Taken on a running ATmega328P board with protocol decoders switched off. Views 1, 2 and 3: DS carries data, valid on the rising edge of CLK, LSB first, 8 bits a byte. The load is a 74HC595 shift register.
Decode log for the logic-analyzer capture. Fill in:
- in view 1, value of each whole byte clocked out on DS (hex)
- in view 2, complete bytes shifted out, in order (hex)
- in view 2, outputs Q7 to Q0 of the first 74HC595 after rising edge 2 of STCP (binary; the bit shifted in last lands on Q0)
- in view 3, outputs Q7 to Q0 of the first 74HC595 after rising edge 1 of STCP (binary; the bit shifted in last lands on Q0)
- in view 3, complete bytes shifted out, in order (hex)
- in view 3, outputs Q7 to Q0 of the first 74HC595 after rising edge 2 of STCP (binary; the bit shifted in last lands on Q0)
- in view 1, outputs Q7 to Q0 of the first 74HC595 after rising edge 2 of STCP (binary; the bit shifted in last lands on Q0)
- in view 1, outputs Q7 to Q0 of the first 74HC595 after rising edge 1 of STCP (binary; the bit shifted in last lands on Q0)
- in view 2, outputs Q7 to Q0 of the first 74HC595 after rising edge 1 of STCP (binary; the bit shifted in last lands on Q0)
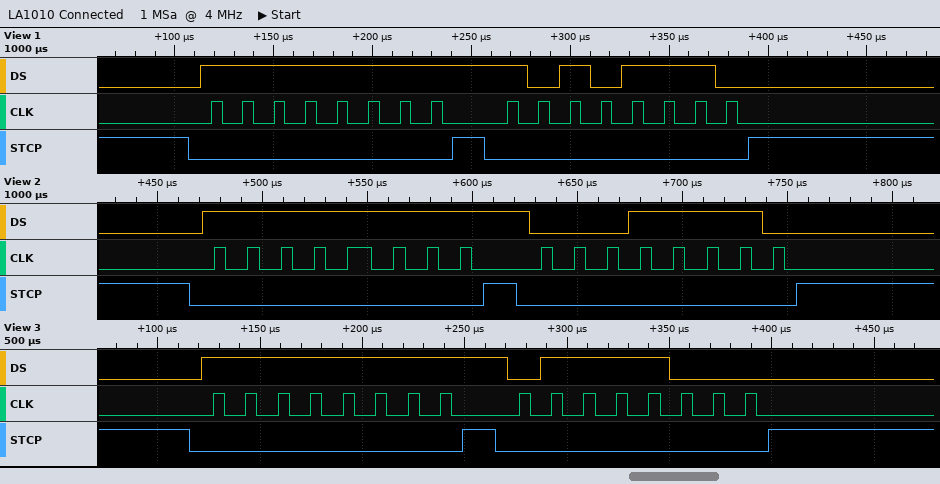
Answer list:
FF 75
0xFF 0x78
00011110
11111111
FF 1E
01111000
10101110
11111111
11111111
